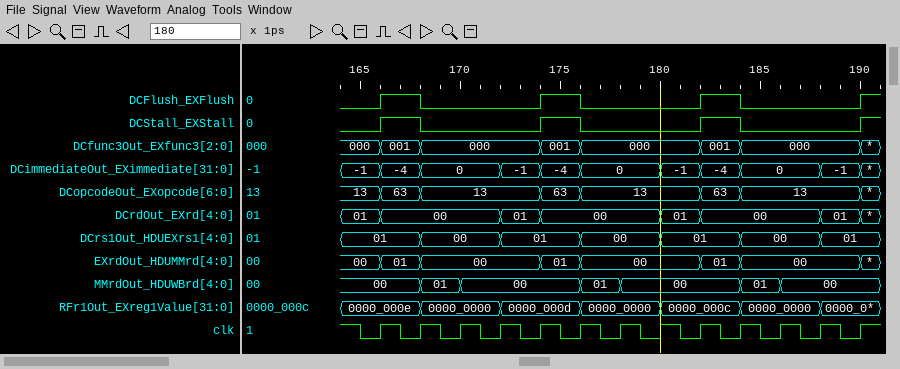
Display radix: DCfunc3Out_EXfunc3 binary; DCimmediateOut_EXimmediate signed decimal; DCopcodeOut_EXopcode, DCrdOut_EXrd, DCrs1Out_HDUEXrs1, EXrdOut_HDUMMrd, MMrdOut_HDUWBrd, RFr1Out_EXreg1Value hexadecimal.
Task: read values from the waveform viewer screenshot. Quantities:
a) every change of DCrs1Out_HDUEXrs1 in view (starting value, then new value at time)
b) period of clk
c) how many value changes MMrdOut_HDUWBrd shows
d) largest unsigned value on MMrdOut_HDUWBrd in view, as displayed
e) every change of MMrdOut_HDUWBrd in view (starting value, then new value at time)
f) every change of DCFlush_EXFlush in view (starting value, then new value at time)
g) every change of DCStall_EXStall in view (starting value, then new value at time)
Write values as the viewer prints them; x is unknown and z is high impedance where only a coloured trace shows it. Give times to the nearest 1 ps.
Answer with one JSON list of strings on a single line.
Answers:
["01, 00 at 168 ps, 01 at 172 ps, 00 at 176 ps, 01 at 180 ps, 00 at 184 ps, 01 at 188 ps", "2 ps", "6", "01", "00, 01 at 168 ps, 00 at 170 ps, 01 at 176 ps, 00 at 178 ps, 01 at 184 ps, 00 at 186 ps", "0, 1 at 166 ps, 0 at 168 ps, 1 at 174 ps, 0 at 176 ps, 1 at 182 ps, 0 at 184 ps, 1 at 190 ps", "0, 1 at 166 ps, 0 at 168 ps, 1 at 174 ps, 0 at 176 ps, 1 at 182 ps, 0 at 184 ps, 1 at 190 ps"]
